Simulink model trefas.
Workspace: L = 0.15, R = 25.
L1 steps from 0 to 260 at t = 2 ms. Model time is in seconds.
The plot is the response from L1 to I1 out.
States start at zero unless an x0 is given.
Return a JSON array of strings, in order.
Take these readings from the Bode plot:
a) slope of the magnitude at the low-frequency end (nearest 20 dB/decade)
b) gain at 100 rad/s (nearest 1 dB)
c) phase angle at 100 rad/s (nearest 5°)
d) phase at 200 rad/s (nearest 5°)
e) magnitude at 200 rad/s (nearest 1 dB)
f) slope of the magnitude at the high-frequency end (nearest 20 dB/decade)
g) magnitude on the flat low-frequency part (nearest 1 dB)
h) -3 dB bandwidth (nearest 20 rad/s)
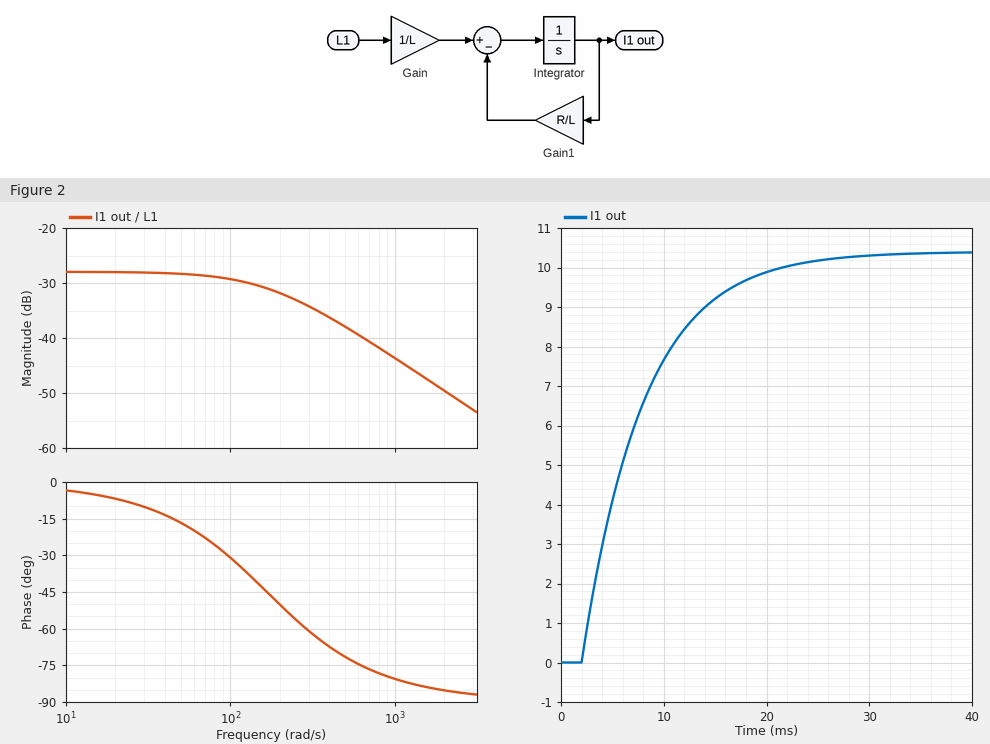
["0 dB/decade", "-29 dB", "-30°", "-50°", "-32 dB", "-20 dB/decade", "-28 dB", "160 rad/s"]
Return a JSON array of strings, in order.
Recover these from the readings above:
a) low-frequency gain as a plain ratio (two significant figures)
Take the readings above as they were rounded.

["0.040"]
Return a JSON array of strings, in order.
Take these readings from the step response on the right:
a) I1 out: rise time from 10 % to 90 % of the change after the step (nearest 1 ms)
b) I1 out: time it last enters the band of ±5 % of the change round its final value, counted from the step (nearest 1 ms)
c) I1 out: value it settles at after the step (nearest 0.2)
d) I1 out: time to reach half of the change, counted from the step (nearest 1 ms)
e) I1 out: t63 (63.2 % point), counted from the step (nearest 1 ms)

["13 ms", "18 ms", "10.4", "4 ms", "6 ms"]
